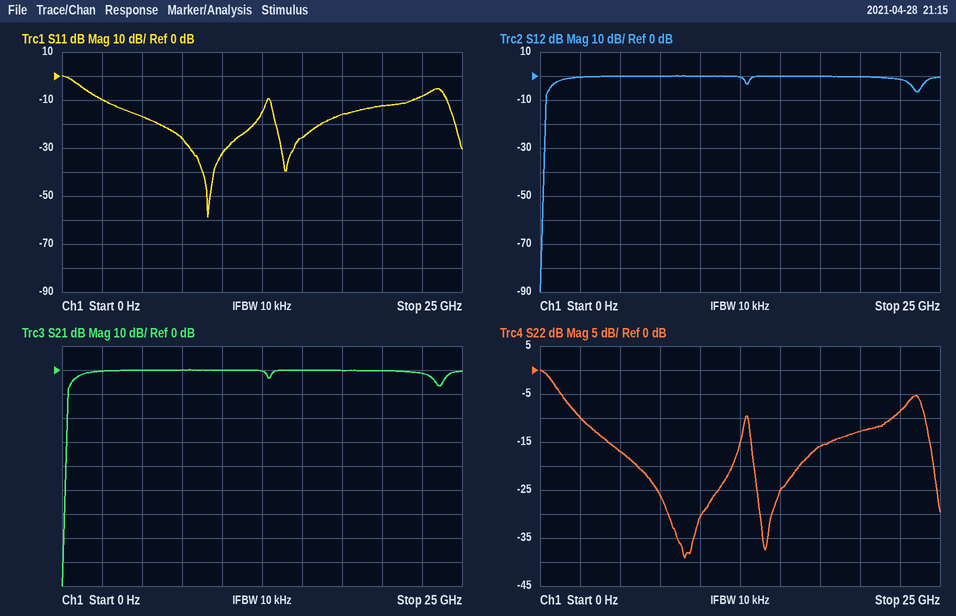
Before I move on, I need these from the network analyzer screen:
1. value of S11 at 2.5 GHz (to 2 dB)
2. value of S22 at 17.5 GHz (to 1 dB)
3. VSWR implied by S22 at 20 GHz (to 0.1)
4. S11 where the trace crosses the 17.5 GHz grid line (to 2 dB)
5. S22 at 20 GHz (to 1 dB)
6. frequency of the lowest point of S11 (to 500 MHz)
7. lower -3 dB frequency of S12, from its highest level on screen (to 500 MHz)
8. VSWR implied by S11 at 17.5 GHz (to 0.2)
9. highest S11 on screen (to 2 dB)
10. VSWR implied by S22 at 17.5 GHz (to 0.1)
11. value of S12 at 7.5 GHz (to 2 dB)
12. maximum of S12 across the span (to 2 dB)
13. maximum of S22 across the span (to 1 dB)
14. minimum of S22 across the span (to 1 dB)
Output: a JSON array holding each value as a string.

["-10 dB", "-16 dB", "1.6", "-16 dB", "-13 dB", "9.0 GHz", "1.0 GHz", "1.4", "0 dB", "1.4", "0 dB", "0 dB", "0 dB", "-39 dB"]
